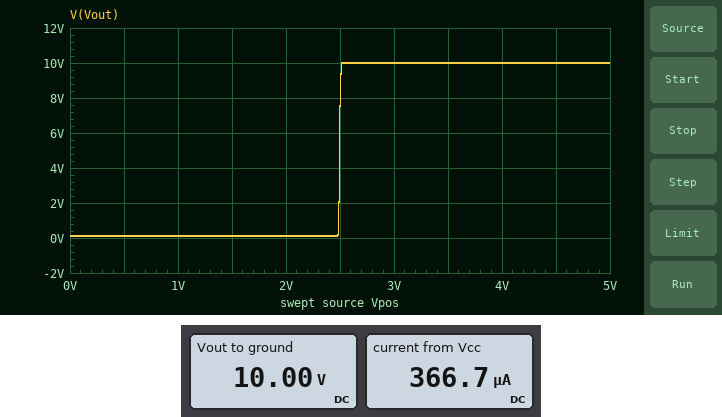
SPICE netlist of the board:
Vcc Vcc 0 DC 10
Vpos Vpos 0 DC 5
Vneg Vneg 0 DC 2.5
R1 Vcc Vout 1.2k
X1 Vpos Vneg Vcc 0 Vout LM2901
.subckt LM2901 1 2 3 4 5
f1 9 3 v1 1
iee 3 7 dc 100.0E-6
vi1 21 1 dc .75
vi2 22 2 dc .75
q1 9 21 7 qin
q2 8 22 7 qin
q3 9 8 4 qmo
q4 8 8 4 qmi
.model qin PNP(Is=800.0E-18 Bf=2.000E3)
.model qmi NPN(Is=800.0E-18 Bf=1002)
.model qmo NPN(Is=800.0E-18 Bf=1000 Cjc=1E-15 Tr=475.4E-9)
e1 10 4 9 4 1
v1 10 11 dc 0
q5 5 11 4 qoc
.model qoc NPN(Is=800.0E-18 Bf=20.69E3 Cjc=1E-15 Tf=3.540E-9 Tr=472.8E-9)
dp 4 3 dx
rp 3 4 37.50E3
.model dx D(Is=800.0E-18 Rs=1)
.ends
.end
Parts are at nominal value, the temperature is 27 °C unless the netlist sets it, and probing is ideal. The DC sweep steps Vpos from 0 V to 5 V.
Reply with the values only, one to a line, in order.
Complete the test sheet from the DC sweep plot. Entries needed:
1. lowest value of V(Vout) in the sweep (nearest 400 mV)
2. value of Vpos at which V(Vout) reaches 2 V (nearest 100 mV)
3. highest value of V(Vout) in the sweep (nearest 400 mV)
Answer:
0 V
2.5 V
10.0 V
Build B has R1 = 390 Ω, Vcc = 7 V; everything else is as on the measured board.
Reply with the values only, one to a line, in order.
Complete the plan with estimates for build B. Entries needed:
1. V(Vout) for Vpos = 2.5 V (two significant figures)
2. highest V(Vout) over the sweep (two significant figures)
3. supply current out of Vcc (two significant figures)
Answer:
6.2 V
7.0 V
290 µA
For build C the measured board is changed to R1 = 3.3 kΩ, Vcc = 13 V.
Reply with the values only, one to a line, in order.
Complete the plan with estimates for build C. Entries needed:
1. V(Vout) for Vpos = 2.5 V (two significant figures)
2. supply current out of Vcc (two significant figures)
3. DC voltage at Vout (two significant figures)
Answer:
6.2 V
450 µA
13 V
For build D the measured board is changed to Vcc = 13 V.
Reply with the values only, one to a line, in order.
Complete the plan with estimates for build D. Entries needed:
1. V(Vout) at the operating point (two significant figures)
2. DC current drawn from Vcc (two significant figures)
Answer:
13 V
450 µA
